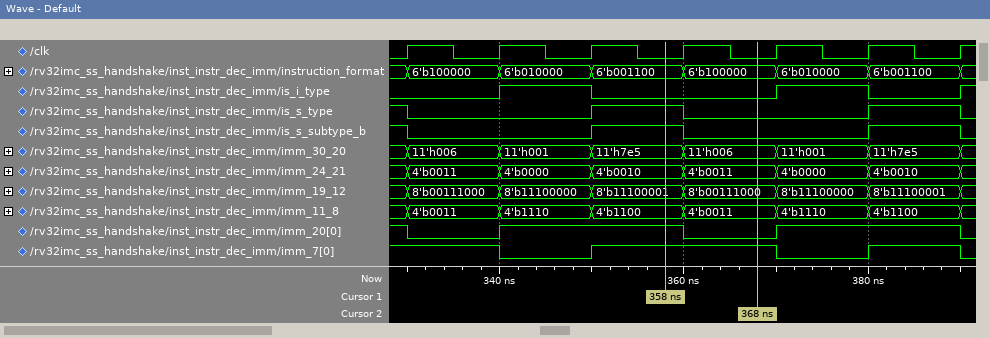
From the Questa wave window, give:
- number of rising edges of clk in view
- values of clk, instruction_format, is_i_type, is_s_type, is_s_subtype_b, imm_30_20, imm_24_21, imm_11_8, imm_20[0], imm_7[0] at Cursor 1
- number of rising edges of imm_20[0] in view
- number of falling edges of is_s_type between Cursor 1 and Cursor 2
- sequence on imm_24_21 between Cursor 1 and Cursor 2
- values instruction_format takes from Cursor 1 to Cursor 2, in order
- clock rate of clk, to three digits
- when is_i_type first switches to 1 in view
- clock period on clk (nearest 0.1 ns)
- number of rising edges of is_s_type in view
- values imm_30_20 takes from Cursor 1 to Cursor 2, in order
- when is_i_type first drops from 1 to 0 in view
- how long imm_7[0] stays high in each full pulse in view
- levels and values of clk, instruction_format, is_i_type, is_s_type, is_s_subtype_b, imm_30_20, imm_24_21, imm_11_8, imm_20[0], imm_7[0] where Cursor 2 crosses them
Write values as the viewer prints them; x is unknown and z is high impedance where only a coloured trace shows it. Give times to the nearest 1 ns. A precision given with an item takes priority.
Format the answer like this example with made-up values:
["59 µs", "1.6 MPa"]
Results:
["7", "clk=0, instruction_format=6'b001100, is_i_type=0, is_s_type=1, is_s_subtype_b=1, imm_30_20=11'h7e5, imm_24_21=4'b0010, imm_11_8=4'b1100, imm_20[0]=1, imm_7[0]=1", "2", "1", "4'b0010, 4'b0011", "6'b001100, 6'b100000", "100 MHz", "340 ns", "10 ns", "2", "11'h7e5, 11'h006", "350 ns", "20 ns, 10 ns", "clk=0, instruction_format=6'b100000, is_i_type=0, is_s_type=0, is_s_subtype_b=0, imm_30_20=11'h006, imm_24_21=4'b0011, imm_11_8=4'b0011, imm_20[0]=0, imm_7[0]=1"]
